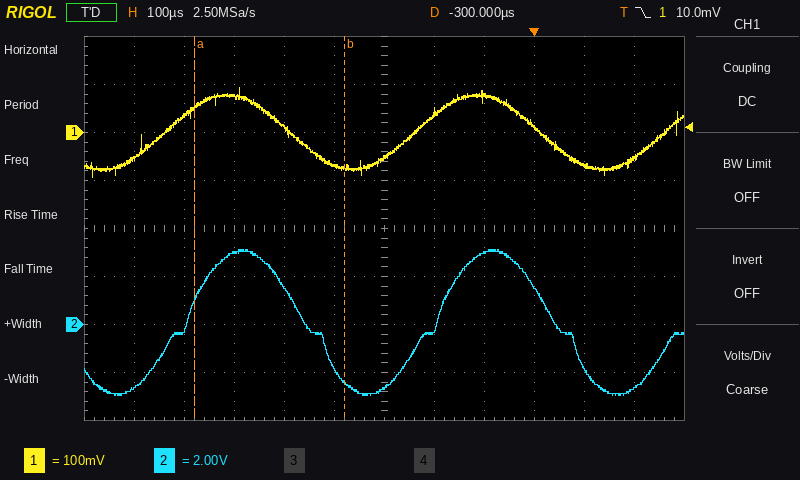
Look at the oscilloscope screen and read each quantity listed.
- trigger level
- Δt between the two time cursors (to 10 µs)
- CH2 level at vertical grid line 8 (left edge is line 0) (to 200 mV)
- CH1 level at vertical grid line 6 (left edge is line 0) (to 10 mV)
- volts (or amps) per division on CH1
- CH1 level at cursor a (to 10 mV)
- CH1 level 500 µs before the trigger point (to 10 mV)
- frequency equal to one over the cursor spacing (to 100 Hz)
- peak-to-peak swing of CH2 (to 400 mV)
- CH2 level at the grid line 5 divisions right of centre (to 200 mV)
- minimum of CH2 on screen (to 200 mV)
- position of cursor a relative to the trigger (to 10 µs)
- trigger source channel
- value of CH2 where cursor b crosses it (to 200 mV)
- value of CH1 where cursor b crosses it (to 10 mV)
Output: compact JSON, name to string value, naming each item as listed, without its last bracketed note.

{"trigger level": "10.0 mV", "Δt between the two time cursors": "300 µs", "CH2 level at vertical grid line 8 (left edge is line 0)": "3.0 V", "CH1 level at vertical grid line 6 (left edge is line 0)": "-50 mV", "volts (or amps) per division on CH1": "100 mV", "CH1 level at cursor a": "50 mV", "CH1 level 500 µs before the trigger point": "10 mV", "frequency equal to one over the cursor spacing": "3.3 kHz", "peak-to-peak swing of CH2": "6.0 V", "CH2 level at the grid line 5 divisions right of centre": "-2.6 V", "minimum of CH2 on screen": "-3.0 V", "position of cursor a relative to the trigger": "-680 µs", "trigger source channel": "CH1", "value of CH2 where cursor b crosses it": "-2.4 V", "value of CH1 where cursor b crosses it": "-70 mV"}
